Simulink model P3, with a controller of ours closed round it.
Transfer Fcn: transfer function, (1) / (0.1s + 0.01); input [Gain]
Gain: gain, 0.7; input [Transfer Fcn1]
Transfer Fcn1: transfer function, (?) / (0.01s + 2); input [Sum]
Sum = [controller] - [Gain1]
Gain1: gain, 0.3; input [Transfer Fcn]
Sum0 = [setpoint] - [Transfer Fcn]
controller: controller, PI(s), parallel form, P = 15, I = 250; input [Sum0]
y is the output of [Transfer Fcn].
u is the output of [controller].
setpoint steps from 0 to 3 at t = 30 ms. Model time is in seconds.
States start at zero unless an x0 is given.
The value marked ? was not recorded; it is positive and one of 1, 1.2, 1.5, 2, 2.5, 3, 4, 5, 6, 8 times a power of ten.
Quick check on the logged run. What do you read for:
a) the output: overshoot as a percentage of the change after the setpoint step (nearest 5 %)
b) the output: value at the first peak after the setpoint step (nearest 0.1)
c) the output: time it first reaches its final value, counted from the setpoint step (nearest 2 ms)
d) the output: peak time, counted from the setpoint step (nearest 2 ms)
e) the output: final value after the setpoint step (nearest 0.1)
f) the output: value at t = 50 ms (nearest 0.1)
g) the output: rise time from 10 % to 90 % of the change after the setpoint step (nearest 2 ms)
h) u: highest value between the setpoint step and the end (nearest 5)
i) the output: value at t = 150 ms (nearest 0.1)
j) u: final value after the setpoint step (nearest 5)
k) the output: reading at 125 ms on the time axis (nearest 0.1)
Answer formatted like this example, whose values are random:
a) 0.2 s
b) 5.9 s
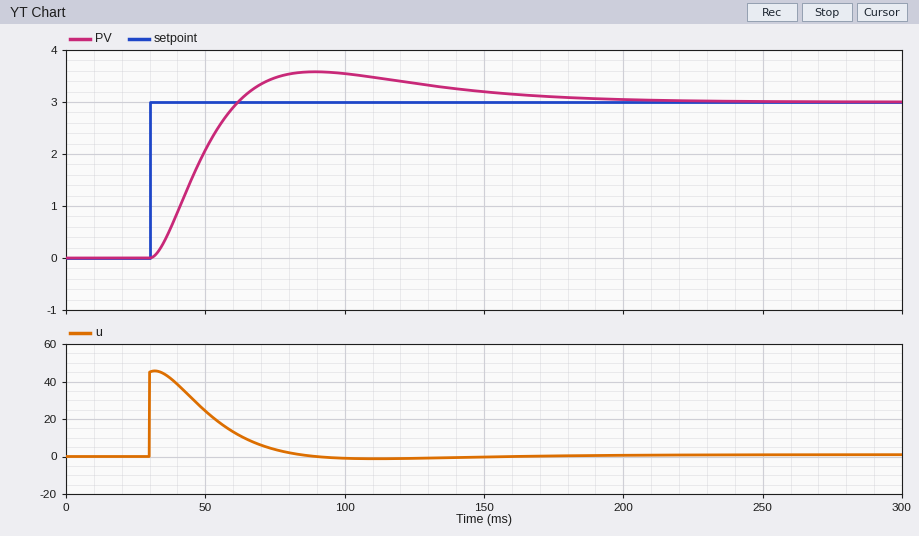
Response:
a) 20 %
b) 3.6
c) 32 ms
d) 60 ms
e) 3.0
f) 2.1
g) 22 ms
h) 45
i) 3.2
j) 0
k) 3.4
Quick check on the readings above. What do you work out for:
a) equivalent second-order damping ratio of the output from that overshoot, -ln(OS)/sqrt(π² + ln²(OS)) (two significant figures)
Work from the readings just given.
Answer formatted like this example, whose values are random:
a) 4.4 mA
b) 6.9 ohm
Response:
a) 0.46
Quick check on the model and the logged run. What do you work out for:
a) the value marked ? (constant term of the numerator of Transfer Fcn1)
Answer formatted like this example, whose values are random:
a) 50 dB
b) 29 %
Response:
a) 1
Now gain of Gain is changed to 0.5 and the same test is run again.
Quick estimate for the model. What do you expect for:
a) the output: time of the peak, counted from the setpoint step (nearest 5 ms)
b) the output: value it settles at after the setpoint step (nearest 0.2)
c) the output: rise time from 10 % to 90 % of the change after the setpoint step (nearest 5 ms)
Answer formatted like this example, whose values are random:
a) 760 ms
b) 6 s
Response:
a) 80 ms
b) 3.0
c) 30 ms
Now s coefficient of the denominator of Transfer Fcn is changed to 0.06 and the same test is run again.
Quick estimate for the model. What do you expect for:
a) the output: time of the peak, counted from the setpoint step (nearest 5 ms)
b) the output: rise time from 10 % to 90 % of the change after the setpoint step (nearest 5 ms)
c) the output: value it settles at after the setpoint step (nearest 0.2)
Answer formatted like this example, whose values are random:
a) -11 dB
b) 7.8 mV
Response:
a) 35 ms
b) 15 ms
c) 3.0
